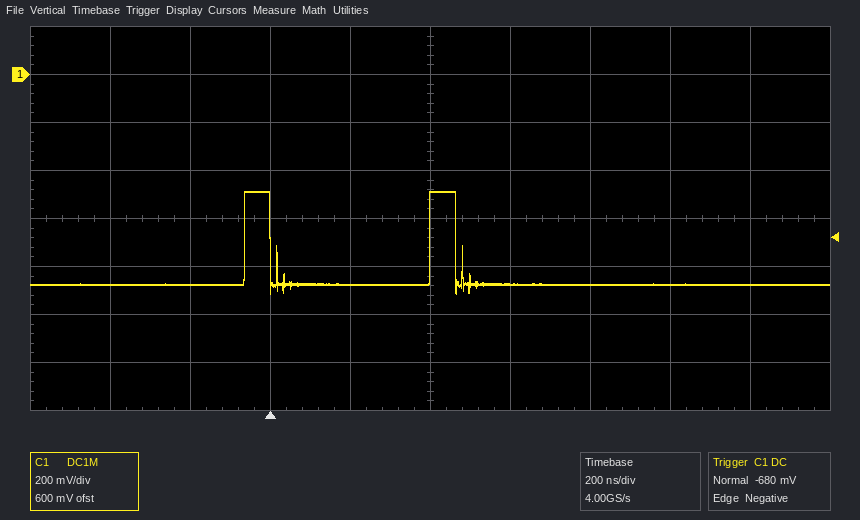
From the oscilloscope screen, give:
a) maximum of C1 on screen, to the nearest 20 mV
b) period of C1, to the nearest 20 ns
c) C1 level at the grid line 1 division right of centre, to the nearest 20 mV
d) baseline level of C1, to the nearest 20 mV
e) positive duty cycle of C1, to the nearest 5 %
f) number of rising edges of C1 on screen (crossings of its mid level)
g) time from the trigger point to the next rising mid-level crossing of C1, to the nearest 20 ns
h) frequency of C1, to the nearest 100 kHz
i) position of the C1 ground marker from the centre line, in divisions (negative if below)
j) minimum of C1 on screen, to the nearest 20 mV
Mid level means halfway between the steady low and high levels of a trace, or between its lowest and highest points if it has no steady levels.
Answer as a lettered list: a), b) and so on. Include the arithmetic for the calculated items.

a) -480 mV
b) 460 ns
c) -880 mV
d) -880 mV
e) 15 %
f) 2
g) 400 ns
h) 1 / 460 ns ≈ 2.2 MHz
i) +3.0 div
j) -920 mV
